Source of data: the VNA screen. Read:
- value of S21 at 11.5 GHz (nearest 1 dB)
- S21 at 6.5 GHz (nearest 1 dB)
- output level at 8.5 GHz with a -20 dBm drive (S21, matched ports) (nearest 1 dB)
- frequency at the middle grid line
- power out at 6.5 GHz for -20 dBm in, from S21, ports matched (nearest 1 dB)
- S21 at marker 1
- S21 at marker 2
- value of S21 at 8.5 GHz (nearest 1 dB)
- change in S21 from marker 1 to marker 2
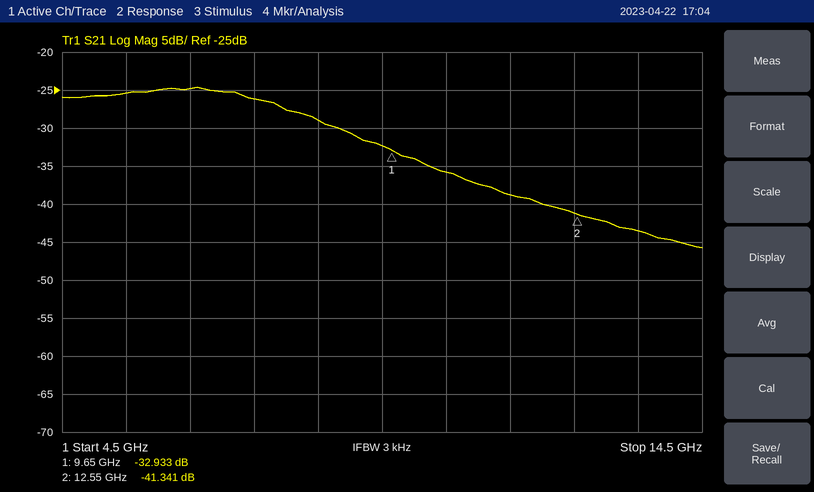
-39 dB
-25 dB
-49 dBm
9.5 GHz
-45 dBm
-32.933 dB
-41.341 dB
-29 dB
-8.408 dB
